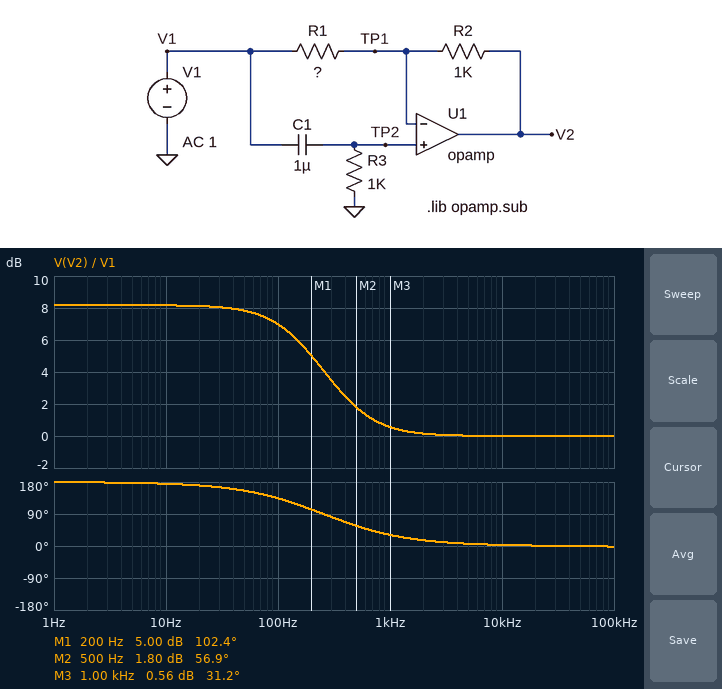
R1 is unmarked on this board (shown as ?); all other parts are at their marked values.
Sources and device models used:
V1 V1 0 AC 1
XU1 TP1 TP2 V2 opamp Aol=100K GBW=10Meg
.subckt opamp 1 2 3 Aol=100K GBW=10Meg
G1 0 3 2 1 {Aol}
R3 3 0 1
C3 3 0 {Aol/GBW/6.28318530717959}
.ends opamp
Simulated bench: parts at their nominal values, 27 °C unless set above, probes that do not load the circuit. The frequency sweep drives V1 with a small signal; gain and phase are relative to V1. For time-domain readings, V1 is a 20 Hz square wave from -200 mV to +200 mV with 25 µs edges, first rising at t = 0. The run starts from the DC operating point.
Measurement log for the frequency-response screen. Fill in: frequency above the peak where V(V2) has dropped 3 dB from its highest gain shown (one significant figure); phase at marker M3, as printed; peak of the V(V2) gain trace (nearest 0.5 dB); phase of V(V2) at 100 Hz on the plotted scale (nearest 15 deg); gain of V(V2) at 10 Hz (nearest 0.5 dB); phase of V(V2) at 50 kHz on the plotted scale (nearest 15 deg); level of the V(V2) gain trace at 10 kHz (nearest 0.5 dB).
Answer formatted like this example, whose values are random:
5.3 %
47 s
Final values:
200 Hz
31.2 deg
8.0 dB
135 deg
8.0 dB
0 deg
0 dB
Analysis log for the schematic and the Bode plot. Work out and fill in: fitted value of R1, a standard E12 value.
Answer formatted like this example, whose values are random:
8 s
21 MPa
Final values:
390 Ω
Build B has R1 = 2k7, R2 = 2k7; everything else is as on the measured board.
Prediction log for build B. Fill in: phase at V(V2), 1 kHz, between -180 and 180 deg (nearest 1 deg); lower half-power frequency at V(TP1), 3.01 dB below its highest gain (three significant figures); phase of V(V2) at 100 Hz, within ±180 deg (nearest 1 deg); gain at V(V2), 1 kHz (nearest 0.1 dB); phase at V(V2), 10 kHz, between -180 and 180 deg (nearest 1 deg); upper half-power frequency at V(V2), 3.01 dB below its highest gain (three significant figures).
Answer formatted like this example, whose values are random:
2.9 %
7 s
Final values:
18 deg
159 Hz
116 deg
0 dB
2 deg
5.00 MHz
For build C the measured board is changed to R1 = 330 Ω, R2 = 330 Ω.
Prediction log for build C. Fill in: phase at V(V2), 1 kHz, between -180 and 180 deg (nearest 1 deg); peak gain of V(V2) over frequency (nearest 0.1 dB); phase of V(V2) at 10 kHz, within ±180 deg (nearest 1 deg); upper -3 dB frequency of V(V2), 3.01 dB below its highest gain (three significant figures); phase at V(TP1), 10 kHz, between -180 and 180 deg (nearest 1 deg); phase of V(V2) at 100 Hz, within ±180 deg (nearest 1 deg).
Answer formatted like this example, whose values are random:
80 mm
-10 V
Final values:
18 deg
0 dB
2 deg
5.00 MHz
1 deg
116 deg
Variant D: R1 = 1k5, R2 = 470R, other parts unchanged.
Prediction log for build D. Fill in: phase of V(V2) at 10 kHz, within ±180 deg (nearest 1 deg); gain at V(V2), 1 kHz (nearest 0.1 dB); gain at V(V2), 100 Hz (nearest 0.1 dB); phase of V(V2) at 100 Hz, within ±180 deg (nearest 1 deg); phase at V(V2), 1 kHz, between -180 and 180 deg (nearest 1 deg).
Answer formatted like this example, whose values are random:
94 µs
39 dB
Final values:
1 deg
-0.1 dB
-4.5 dB
84 deg
12 deg
